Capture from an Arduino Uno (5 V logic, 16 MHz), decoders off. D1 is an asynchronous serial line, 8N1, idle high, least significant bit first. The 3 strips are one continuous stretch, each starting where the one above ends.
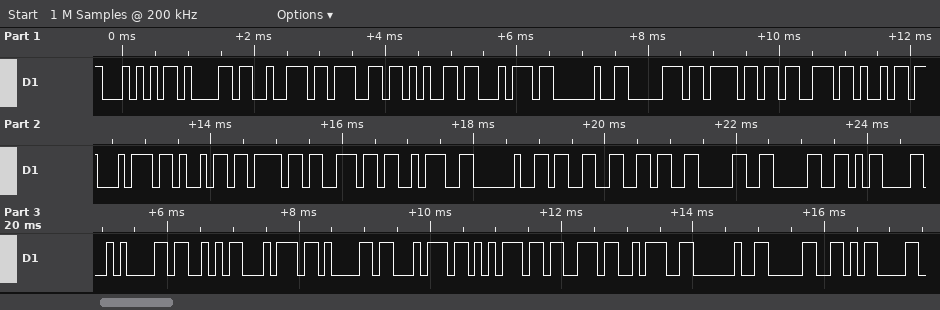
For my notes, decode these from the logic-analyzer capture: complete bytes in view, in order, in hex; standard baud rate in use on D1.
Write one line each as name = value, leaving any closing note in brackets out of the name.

complete bytes in view, in order, in hex = 54 61 72 67 65 74 20 70 6F 73 69 74 69 6F 6E 3A 20 33 36 30 30 0D 0A 53 74 61 74 75 73 3A 20 30 0D
standard baud rate in use on D1 = 9600 baud
